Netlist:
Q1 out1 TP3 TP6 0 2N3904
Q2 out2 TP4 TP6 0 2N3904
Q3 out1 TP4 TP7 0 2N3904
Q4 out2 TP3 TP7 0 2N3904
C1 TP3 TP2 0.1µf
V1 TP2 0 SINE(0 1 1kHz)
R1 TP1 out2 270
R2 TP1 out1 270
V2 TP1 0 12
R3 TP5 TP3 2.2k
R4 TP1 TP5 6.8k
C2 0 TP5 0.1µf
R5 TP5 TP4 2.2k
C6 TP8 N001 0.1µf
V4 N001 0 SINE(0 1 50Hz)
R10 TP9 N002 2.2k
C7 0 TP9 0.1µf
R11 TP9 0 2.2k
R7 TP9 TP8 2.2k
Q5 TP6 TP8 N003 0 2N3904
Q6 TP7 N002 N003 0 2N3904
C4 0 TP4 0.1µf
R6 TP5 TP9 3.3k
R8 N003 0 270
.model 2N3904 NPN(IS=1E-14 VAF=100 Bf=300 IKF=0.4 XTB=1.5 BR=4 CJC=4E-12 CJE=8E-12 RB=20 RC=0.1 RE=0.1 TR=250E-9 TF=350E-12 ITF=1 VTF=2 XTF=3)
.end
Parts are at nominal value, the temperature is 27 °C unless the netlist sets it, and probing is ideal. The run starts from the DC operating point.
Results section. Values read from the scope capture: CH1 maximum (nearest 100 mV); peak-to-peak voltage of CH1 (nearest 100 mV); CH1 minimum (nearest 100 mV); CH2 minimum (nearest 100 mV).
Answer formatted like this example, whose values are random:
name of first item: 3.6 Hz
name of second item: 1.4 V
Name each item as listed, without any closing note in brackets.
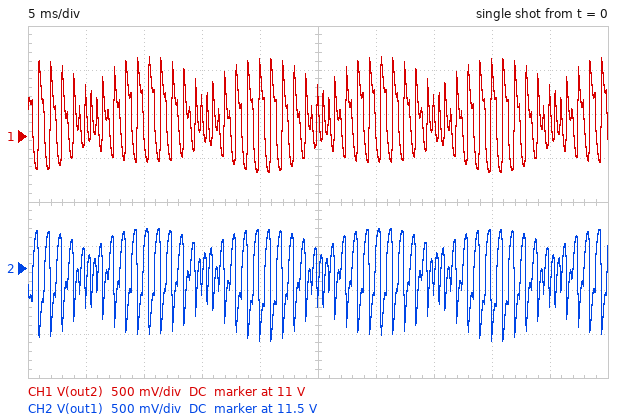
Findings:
CH1 maximum: 11.9 V
peak-to-peak voltage of CH1: 1.3 V
CH1 minimum: 10.6 V
CH2 minimum: 10.7 V
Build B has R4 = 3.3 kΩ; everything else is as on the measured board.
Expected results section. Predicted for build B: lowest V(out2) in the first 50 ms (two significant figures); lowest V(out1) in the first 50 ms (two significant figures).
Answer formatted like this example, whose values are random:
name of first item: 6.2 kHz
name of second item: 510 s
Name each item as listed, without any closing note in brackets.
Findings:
lowest V(out2) in the first 50 ms: 9.9 V
lowest V(out1) in the first 50 ms: 10 V
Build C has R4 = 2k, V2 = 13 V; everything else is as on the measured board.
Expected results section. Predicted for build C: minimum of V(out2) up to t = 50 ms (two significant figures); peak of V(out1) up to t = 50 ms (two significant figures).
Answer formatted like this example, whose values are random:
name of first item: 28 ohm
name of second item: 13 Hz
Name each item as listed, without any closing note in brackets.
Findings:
minimum of V(out2) up to t = 50 ms: 10 V
peak of V(out1) up to t = 50 ms: 13 V
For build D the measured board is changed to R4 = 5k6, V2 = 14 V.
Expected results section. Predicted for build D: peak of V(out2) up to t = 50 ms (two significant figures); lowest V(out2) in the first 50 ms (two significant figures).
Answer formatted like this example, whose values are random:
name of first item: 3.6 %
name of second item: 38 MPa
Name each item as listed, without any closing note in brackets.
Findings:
peak of V(out2) up to t = 50 ms: 14 V
lowest V(out2) in the first 50 ms: 12 V
